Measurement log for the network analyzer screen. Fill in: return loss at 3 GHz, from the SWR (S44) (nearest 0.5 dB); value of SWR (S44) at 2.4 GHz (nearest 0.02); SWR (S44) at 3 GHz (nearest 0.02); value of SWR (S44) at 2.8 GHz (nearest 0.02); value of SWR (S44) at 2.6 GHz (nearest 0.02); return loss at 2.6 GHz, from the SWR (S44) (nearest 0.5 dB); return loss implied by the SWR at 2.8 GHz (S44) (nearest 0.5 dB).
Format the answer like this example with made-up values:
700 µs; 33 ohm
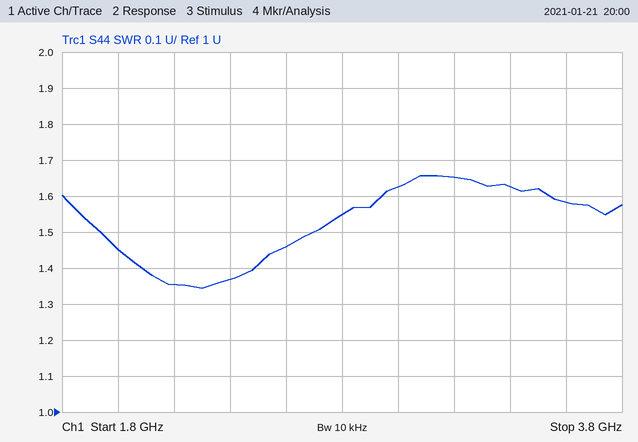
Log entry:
12.5 dB; 1.36; 1.62; 1.54; 1.46; 14.5 dB; 13.5 dB
